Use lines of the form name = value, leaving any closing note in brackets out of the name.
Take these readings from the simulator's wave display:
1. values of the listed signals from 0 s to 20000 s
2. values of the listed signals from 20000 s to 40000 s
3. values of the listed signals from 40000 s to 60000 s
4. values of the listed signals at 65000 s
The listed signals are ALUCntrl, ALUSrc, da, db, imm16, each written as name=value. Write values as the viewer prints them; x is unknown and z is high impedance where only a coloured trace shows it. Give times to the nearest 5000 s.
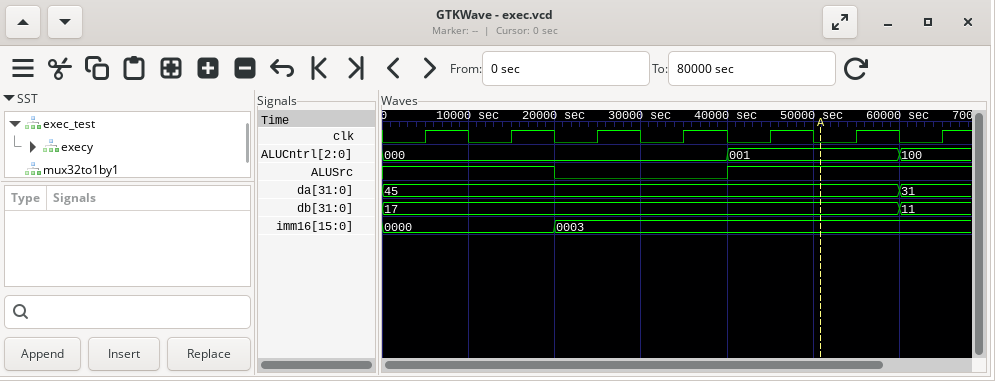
values of the listed signals from 0 s to 20000 s = ALUCntrl=000, ALUSrc=1, da=45, db=17, imm16=0000
values of the listed signals from 20000 s to 40000 s = ALUCntrl=000, ALUSrc=0, da=45, db=17, imm16=0003
values of the listed signals from 40000 s to 60000 s = ALUCntrl=001, ALUSrc=1, da=45, db=17, imm16=0003
values of the listed signals at 65000 s = ALUCntrl=100, ALUSrc=1, da=31, db=11, imm16=0003
